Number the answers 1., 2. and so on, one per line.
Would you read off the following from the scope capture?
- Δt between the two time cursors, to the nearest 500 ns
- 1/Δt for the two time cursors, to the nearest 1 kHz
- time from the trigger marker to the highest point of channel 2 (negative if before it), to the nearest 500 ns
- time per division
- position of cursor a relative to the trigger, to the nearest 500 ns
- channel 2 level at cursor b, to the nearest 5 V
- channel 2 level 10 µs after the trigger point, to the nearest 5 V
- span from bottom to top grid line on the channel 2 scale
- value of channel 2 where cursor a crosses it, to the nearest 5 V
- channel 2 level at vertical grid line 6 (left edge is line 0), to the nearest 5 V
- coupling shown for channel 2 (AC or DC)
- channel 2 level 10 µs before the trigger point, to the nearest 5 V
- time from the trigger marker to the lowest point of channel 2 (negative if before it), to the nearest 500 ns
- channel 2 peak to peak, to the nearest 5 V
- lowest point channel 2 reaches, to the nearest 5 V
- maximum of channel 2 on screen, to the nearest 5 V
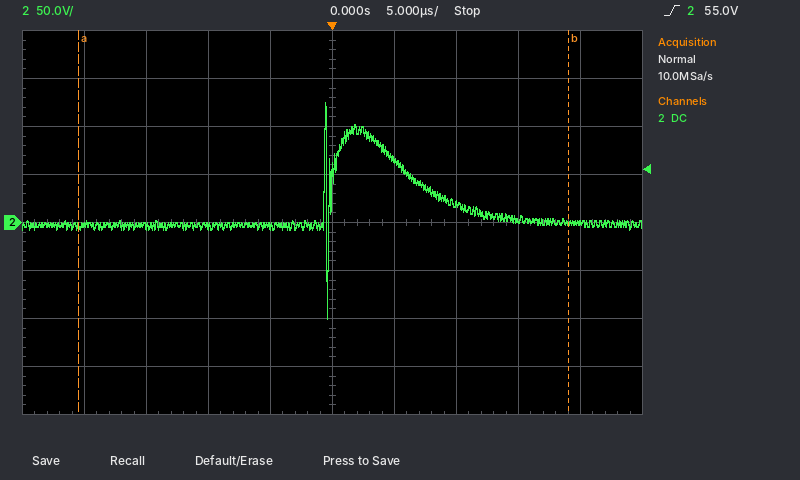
1. 39.5 µs
2. 25 kHz
3. -500 ns
4. 5 µs
5. -20.5 µs
6. 0 V
7. 20 V
8. 400 V
9. -5 V
10. 65 V
11. DC
12. -5 V
13. -500 ns
14. 225 V
15. -100 V
16. 125 V
